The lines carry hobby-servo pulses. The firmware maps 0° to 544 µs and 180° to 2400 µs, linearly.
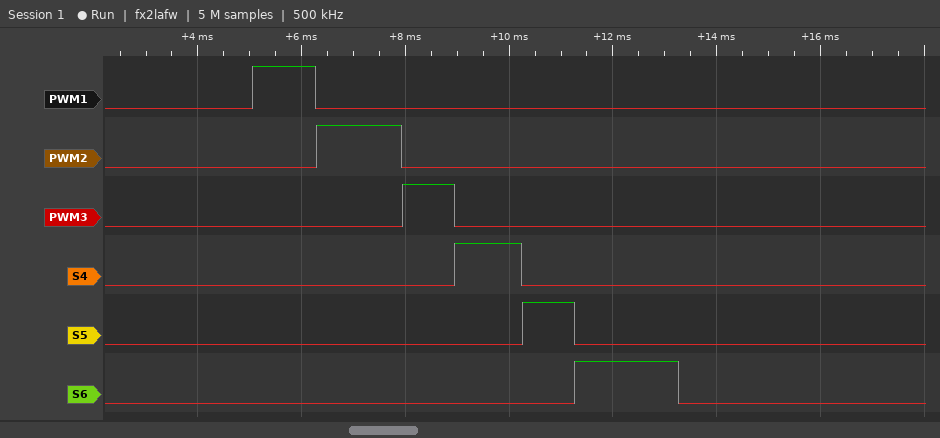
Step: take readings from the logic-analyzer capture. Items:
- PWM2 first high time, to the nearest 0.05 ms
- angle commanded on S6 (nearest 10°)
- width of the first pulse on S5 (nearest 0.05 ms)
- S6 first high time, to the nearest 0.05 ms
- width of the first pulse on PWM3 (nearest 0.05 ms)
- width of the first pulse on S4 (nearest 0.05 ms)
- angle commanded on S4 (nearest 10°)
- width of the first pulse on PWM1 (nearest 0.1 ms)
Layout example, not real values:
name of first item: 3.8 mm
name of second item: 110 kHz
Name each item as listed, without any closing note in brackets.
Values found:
PWM2 first high time, to the nearest 0.05 ms: 1.65 ms
angle commanded on S6: 140°
width of the first pulse on S5: 1.00 ms
S6 first high time, to the nearest 0.05 ms: 2.00 ms
width of the first pulse on PWM3: 1.00 ms
width of the first pulse on S4: 1.30 ms
angle commanded on S4: 70°
width of the first pulse on PWM1: 1.2 ms
